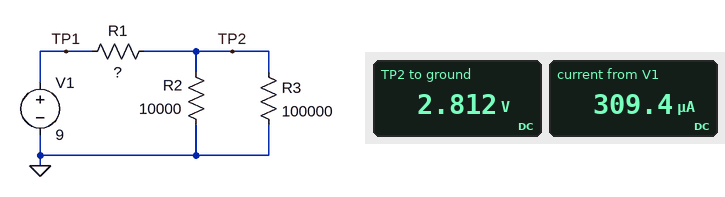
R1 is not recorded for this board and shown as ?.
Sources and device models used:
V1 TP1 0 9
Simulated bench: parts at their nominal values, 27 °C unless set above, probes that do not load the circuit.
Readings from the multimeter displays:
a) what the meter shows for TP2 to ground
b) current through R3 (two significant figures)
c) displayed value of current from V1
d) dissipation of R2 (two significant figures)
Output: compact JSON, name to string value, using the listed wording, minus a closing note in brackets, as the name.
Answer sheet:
{"what the meter shows for TP2 to ground": "2.812 V", "current through R3": "28 µA", "displayed value of current from V1": "309.4 µA", "dissipation of R2": "790 µW"}
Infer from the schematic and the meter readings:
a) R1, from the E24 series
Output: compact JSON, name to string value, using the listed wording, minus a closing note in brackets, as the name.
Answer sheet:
{"R1, from the E24 series": "20 kΩ"}
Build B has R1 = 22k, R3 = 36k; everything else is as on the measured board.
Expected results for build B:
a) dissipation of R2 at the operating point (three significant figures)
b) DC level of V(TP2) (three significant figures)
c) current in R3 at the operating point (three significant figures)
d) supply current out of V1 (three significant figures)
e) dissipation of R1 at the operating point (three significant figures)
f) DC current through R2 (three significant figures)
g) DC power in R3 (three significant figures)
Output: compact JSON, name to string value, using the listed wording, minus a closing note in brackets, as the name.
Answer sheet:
{"dissipation of R2 at the operating point": "558 µW", "DC level of V(TP2)": "2.36 V", "current in R3 at the operating point": "65.6 µA", "supply current out of V1": "302 µA", "dissipation of R1 at the operating point": "2.00 mW", "DC current through R2": "236 µA", "DC power in R3": "155 µW"}
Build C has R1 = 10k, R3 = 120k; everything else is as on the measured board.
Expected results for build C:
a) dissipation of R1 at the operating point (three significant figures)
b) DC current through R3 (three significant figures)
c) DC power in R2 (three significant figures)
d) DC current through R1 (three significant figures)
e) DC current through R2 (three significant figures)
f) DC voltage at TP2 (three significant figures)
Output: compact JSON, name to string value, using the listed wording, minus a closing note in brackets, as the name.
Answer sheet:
{"dissipation of R1 at the operating point": "2.19 mW", "DC current through R3": "36.0 µA", "DC power in R2": "1.87 mW", "DC current through R1": "468 µA", "DC current through R2": "432 µA", "DC voltage at TP2": "4.32 V"}
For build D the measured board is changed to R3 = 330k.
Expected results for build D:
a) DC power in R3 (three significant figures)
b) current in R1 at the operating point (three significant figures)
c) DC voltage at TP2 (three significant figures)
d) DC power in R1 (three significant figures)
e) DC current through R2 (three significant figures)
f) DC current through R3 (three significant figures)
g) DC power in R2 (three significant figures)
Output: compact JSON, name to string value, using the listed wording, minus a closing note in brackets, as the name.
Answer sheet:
{"DC power in R3": "26.2 µW", "current in R1 at the operating point": "303 µA", "DC voltage at TP2": "2.94 V", "DC power in R1": "1.84 mW", "DC current through R2": "294 µA", "DC current through R3": "8.91 µA", "DC power in R2": "865 µW"}
